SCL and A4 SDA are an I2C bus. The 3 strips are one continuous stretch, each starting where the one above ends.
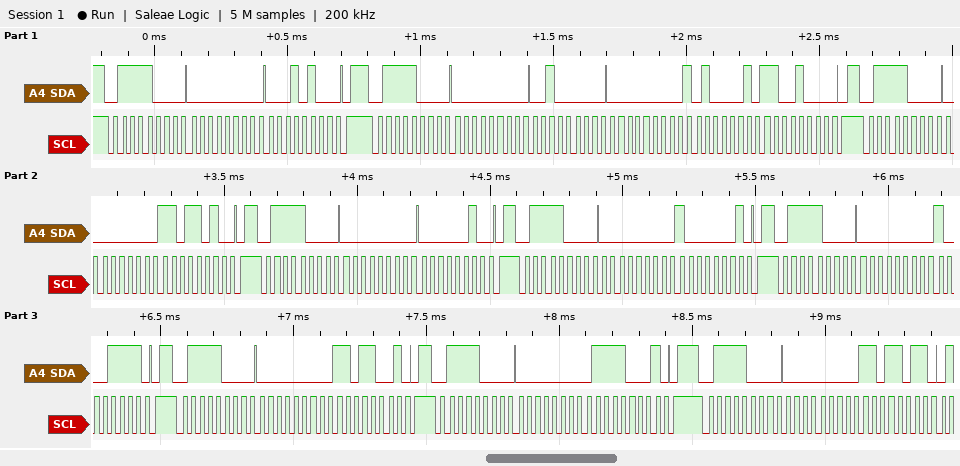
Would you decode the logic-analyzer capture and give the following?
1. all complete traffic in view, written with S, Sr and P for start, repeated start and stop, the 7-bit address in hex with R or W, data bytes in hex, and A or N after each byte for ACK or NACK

S 3CW A 00 A 14 A P S 3CW A 00 A 20 A 00 A A1 A C8 A P S 3CW A 00 A DA A P S 3CW A 00 A 02 A P S 3CW A 00 A 81 A P S 3CW A 00 A 8F A P S 3CW A 00 A D9 A P S 3CW A 00 A F1 A P S 3CW A 00 A DB A
